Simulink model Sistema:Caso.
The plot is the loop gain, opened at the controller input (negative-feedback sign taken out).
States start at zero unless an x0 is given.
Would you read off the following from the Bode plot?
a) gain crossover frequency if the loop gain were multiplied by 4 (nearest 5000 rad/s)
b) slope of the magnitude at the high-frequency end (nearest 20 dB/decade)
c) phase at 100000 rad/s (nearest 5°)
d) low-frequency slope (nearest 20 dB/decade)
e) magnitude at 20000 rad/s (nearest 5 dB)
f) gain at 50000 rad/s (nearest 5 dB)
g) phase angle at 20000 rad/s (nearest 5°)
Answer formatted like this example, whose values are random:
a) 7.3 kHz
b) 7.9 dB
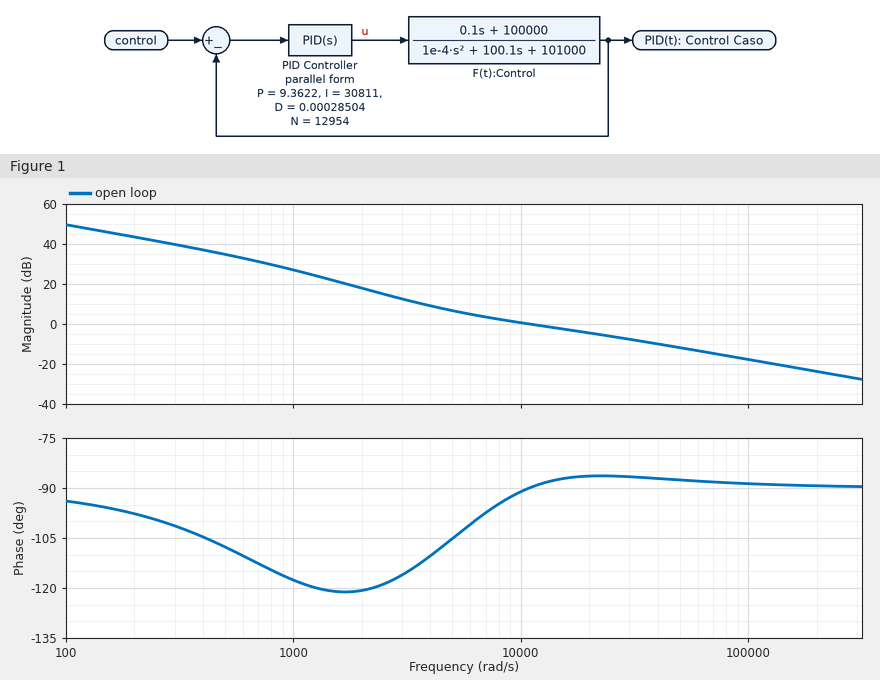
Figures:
a) 50000 rad/s
b) -20 dB/decade
c) -90°
d) -20 dB/decade
e) -5 dB
f) -10 dB
g) -85°
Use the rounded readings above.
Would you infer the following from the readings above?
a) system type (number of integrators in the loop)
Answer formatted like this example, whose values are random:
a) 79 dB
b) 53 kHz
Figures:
a) 1
